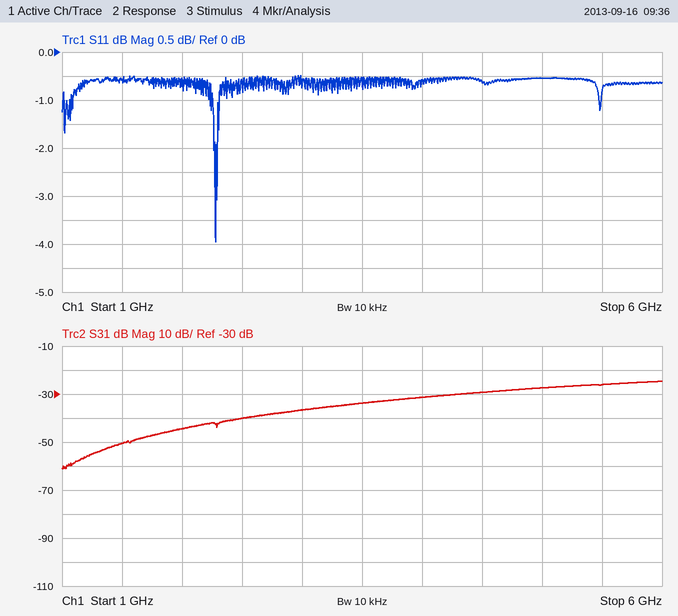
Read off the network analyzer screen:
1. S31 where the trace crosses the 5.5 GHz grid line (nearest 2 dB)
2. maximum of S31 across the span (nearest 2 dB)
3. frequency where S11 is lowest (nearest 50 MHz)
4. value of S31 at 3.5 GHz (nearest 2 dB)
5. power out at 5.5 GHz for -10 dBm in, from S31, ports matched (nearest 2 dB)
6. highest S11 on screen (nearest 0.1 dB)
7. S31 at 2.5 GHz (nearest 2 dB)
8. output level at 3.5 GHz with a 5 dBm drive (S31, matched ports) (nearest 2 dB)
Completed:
-26 dB
-24 dB
2.30 GHz
-34 dB
-36 dBm
-0.5 dB
-40 dB
-28 dBm
